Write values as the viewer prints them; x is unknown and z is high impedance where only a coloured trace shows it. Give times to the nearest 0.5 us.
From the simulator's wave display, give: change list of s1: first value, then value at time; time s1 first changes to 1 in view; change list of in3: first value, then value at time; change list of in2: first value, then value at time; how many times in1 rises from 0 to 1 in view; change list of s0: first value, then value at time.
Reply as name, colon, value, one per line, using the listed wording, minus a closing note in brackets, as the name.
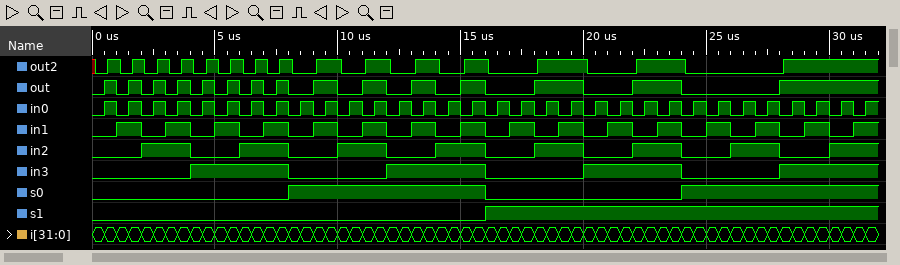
change list of s1: first value, then value at time: 0, 1 at 16 us
time s1 first changes to 1 in view: 16 us
change list of in3: first value, then value at time: 0, 1 at 4 us, 0 at 8 us, 1 at 12 us, 0 at 16 us, 1 at 20 us, 0 at 24 us, 1 at 28 us
change list of in2: first value, then value at time: 0, 1 at 2 us, 0 at 4 us, 1 at 6 us, 0 at 8 us, 1 at 10 us, 0 at 12 us, 1 at 14 us, 0 at 16 us, 1 at 18 us, 0 at 20 us, 1 at 22 us, 0 at 24 us, 1 at 26 us, 0 at 28 us, 1 at 30 us
how many times in1 rises from 0 to 1 in view: 16
change list of s0: first value, then value at time: 0, 1 at 8 us, 0 at 16 us, 1 at 24 us
